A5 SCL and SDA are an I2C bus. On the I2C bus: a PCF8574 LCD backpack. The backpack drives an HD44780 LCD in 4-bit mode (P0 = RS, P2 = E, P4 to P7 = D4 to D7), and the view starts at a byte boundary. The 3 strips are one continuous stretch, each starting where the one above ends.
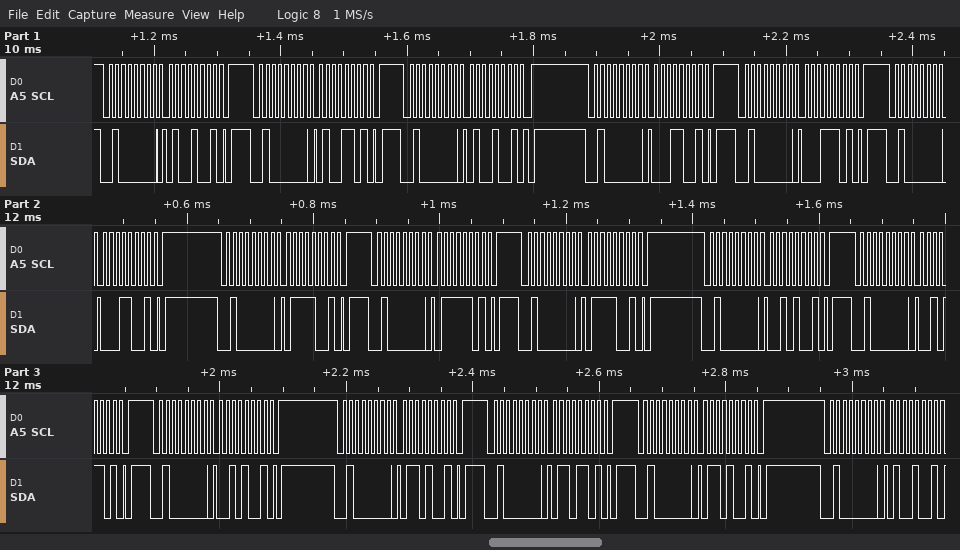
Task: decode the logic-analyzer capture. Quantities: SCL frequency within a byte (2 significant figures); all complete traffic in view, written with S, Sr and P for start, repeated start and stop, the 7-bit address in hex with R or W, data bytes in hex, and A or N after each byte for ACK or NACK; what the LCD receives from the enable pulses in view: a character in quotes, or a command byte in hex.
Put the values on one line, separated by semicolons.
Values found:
100 kHz; S 20W A 49 A P S 20W A 4D A P S 20W A 49 A P S 20W A 19 A P S 20W A 1D A P S 20W A 19 A P S 20W A 79 A P S 20W A 7D A P S 20W A 79 A P S 20W A 29 A P S 20W A 2D A P S 20W A 29 A P S 20W A 69 A P S 20W A 6D A P S 20W A 69 A P S 20W A 49 A; 'A' 'r'
